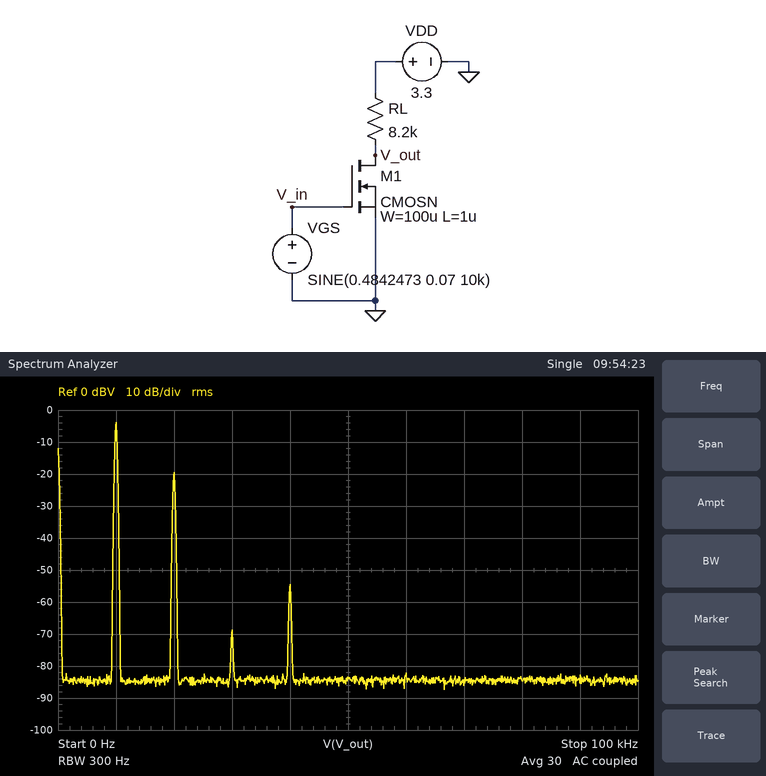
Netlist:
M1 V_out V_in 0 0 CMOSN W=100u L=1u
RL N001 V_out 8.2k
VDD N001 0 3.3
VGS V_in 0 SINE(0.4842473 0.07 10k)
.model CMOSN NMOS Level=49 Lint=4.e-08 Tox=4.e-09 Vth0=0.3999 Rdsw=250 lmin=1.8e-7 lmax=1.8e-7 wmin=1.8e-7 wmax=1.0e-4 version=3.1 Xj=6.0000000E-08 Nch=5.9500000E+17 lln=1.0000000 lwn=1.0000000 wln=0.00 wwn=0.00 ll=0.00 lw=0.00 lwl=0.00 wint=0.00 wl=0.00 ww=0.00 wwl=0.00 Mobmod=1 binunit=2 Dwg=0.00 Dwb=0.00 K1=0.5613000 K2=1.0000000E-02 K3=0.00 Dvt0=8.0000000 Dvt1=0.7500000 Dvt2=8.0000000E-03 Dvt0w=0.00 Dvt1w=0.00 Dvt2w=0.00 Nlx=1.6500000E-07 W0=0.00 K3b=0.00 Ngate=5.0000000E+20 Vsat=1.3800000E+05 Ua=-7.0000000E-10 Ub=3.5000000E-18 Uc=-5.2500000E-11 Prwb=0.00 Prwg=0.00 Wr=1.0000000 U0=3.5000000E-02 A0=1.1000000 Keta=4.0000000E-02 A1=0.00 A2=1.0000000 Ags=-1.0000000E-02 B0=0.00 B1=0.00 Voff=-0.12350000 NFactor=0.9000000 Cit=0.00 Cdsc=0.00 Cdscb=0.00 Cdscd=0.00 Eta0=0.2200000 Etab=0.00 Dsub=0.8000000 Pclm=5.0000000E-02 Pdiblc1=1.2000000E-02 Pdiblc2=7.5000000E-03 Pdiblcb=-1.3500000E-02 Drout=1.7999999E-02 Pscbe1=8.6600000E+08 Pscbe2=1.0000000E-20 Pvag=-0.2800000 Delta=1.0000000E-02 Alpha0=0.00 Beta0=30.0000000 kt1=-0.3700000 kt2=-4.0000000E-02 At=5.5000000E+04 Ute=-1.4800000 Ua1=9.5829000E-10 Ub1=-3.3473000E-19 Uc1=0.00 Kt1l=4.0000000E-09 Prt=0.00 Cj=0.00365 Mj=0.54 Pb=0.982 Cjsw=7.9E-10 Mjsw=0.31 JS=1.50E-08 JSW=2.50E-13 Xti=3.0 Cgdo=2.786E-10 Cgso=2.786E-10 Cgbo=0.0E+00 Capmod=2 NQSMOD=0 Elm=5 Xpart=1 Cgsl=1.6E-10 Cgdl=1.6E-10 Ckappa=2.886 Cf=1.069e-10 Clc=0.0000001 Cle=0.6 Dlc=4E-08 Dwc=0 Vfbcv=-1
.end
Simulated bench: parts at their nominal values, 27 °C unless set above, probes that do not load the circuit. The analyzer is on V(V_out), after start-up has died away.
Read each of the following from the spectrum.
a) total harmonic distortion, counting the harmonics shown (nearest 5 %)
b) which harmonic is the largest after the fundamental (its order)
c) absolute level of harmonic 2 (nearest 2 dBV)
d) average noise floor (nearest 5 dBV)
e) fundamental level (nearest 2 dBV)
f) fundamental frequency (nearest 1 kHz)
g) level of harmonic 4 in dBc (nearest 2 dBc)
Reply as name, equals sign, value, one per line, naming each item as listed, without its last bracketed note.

total harmonic distortion, counting the harmonics shown = 15 %
which harmonic is the largest after the fundamental = 2
absolute level of harmonic 2 = -20 dBV
average noise floor = -85 dBV
fundamental level = -4 dBV
fundamental frequency = 10 kHz
level of harmonic 4 in dBc = -50 dBc
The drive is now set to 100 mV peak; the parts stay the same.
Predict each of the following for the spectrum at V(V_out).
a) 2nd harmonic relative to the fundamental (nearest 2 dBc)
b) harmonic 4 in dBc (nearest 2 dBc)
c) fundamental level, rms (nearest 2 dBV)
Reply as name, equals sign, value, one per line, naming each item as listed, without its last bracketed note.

2nd harmonic relative to the fundamental = -14 dBc
harmonic 4 in dBc = -42 dBc
fundamental level, rms = 0 dBV
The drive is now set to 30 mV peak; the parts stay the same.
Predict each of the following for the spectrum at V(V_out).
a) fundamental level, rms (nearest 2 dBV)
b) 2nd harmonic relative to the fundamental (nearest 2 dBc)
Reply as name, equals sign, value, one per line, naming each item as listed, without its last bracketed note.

fundamental level, rms = -12 dBV
2nd harmonic relative to the fundamental = -22 dBc
